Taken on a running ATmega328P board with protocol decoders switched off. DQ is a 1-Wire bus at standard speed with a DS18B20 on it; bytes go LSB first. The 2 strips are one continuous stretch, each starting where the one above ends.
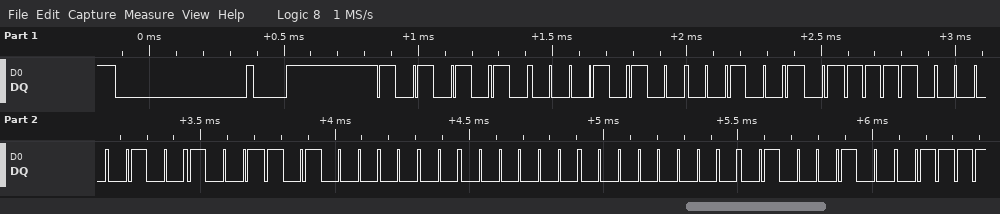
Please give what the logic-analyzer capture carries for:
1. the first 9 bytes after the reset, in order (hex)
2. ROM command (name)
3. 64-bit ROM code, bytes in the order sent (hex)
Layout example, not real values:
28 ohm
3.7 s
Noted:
55 28 A4 0F 92 05 00 00 22
Match ROM
28 A4 0F 92 05 00 00 22
